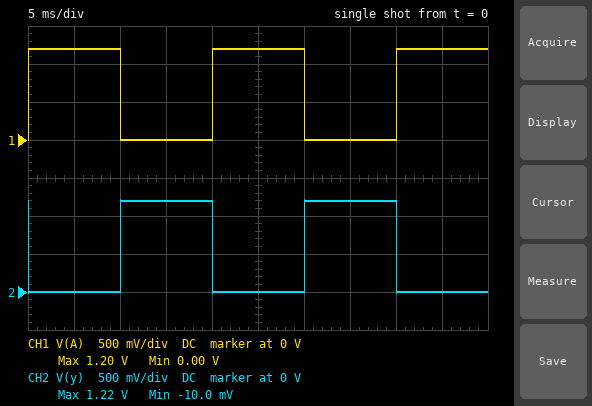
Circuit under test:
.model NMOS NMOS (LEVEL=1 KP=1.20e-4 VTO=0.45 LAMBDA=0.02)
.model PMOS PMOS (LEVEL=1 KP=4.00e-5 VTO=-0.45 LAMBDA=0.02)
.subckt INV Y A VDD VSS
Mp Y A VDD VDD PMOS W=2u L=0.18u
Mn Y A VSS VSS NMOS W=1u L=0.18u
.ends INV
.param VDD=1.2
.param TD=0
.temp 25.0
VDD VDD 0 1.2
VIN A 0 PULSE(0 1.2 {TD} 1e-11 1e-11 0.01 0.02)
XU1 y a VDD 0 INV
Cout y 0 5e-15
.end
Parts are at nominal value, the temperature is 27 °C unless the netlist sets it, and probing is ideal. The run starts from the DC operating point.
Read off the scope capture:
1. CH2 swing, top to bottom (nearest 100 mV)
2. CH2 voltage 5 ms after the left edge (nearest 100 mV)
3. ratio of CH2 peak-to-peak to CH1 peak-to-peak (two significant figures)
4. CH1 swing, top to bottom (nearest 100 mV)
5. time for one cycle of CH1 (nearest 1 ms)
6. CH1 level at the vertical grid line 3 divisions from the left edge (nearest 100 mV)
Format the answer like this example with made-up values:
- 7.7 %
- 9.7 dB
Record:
- 1.2 V
- 0 V
- 1.0
- 1.2 V
- 20 ms
- 0 V
